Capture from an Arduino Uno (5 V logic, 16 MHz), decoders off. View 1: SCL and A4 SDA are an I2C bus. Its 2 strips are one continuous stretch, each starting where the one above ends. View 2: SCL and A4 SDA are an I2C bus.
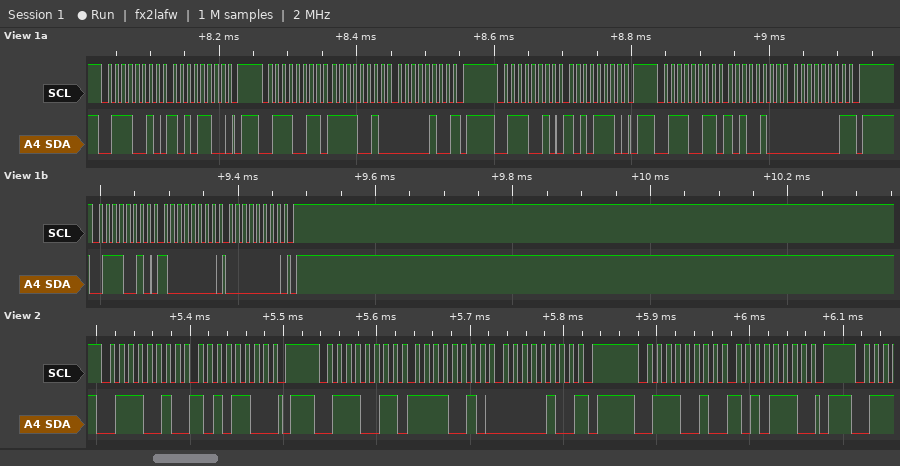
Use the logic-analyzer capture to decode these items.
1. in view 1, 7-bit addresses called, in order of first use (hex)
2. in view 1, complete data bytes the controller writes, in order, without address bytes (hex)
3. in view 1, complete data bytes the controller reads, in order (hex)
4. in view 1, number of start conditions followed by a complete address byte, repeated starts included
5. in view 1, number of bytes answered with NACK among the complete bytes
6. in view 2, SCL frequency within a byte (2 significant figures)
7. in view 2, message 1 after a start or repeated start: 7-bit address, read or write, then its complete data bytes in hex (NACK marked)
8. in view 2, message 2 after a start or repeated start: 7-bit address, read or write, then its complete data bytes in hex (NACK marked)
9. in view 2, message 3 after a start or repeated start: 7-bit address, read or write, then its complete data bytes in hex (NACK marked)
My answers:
0x39
AC AE 80 00
F2 04 A4 01
5
2
100 kHz
0x39 write: AC
0x39 read: F2 04 NACK
0x39 write: AE
